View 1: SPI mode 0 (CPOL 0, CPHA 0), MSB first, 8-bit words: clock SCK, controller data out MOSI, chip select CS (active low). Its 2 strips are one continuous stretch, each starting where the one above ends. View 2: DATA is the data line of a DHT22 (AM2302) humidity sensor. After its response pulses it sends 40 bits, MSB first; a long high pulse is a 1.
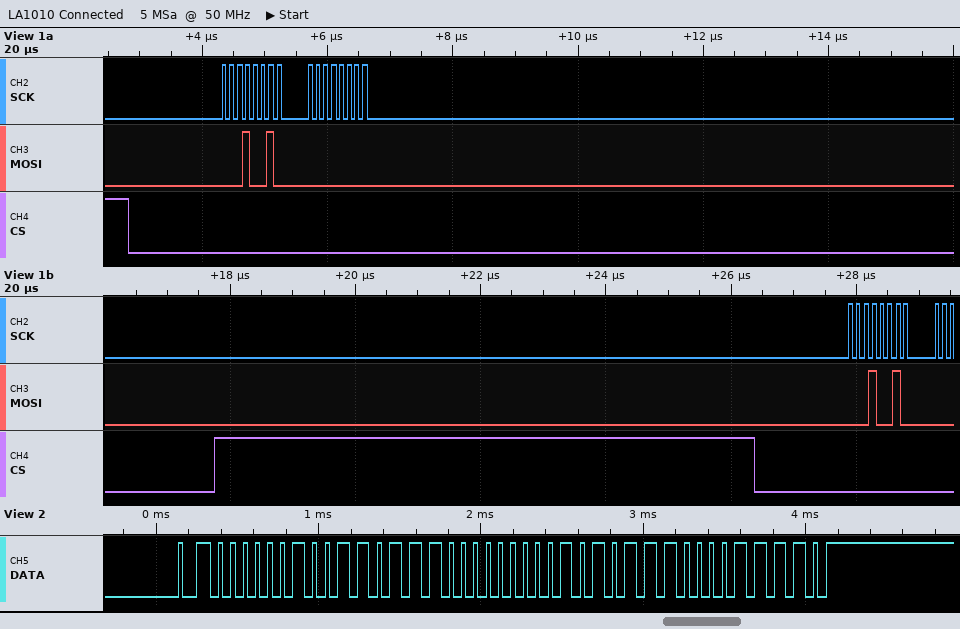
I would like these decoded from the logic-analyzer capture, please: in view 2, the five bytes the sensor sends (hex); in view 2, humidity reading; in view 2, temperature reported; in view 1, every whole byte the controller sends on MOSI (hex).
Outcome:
02 6E 00 AE 1E
62.2 %
17.4 °C
12 00 12
